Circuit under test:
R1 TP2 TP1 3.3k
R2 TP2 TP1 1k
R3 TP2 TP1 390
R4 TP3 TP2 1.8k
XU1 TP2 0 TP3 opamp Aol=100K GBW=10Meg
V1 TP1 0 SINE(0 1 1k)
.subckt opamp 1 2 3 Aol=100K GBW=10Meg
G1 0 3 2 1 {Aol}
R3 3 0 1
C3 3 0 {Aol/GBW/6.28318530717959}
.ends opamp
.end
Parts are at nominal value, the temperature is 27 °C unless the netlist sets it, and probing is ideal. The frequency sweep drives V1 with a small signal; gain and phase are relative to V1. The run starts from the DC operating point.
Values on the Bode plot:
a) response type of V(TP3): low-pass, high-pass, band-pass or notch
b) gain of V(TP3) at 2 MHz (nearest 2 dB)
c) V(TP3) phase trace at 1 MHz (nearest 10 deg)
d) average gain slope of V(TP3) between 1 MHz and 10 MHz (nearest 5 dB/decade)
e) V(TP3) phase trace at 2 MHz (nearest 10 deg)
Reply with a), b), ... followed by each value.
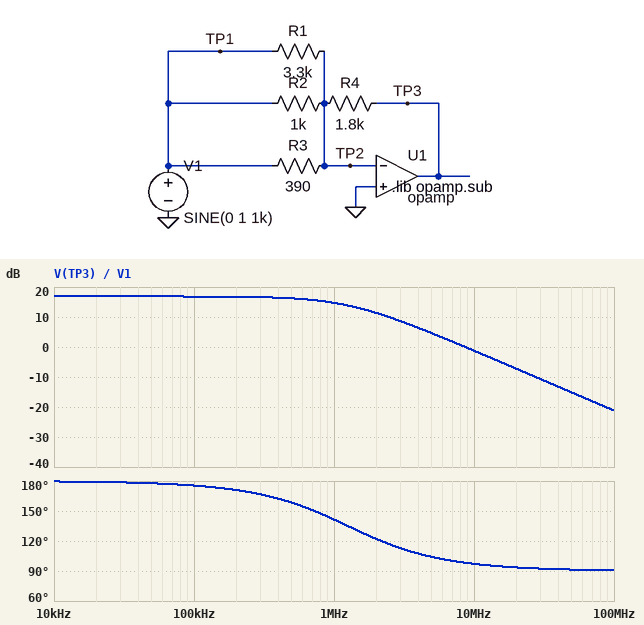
a) low-pass
b) 12 dB
c) 140 deg
d) -15 dB/decade
e) 120 deg
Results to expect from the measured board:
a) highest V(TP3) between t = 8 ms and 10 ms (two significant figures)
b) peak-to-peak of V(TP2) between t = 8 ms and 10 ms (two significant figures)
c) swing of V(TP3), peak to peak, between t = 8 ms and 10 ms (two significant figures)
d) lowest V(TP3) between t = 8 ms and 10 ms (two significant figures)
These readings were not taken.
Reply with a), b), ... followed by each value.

a) 7.0 V
b) 1.4 mV
c) 14 V
d) -7.0 V
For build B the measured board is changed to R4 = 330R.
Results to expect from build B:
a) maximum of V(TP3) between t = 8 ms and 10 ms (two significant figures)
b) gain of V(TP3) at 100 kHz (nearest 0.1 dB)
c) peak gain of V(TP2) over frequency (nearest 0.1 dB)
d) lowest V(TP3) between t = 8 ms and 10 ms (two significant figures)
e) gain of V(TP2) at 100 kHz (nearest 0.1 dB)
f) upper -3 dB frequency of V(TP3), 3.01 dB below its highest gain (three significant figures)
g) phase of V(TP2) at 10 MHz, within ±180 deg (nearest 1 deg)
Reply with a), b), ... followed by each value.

a) 1.3 V
b) 2.1 dB
c) -5.0 dB
d) -1.3 V
e) -37.9 dB
f) 4.39 MHz
g) 24 deg
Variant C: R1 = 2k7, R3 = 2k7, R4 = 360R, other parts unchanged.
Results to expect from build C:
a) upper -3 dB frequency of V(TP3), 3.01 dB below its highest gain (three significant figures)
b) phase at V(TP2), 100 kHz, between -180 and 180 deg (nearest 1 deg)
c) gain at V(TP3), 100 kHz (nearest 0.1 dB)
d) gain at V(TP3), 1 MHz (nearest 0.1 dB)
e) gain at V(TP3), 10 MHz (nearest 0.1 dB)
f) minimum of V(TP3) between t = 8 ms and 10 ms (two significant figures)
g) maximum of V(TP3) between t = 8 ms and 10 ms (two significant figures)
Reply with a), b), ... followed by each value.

a) 6.15 MHz
b) 89 deg
c) -4.1 dB
d) -4.2 dB
e) -9.7 dB
f) -630 mV
g) 630 mV
